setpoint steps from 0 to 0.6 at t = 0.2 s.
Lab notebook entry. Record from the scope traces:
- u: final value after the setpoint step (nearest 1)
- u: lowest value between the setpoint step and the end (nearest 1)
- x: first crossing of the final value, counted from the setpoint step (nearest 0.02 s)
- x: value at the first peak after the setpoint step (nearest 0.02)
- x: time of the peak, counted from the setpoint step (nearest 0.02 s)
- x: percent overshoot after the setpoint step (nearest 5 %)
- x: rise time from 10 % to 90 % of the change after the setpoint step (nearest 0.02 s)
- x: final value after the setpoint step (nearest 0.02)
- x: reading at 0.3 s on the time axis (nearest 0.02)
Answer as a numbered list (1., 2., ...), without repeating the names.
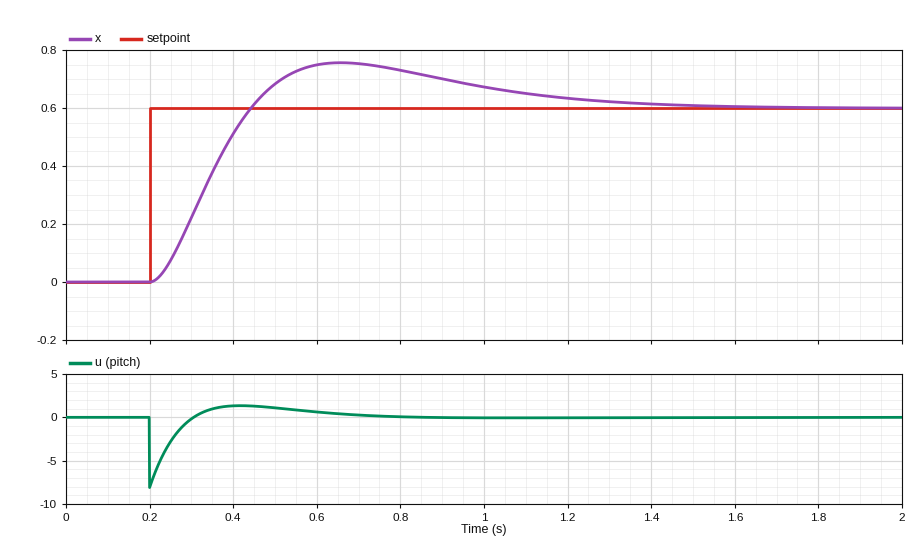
1. 0
2. -8
3. 0.24 s
4. 0.76
5. 0.46 s
6. 25 %
7. 0.16 s
8. 0.60
9. 0.22
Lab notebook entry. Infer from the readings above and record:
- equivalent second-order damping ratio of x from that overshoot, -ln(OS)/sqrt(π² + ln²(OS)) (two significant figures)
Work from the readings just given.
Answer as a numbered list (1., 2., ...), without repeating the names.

1. 0.40
